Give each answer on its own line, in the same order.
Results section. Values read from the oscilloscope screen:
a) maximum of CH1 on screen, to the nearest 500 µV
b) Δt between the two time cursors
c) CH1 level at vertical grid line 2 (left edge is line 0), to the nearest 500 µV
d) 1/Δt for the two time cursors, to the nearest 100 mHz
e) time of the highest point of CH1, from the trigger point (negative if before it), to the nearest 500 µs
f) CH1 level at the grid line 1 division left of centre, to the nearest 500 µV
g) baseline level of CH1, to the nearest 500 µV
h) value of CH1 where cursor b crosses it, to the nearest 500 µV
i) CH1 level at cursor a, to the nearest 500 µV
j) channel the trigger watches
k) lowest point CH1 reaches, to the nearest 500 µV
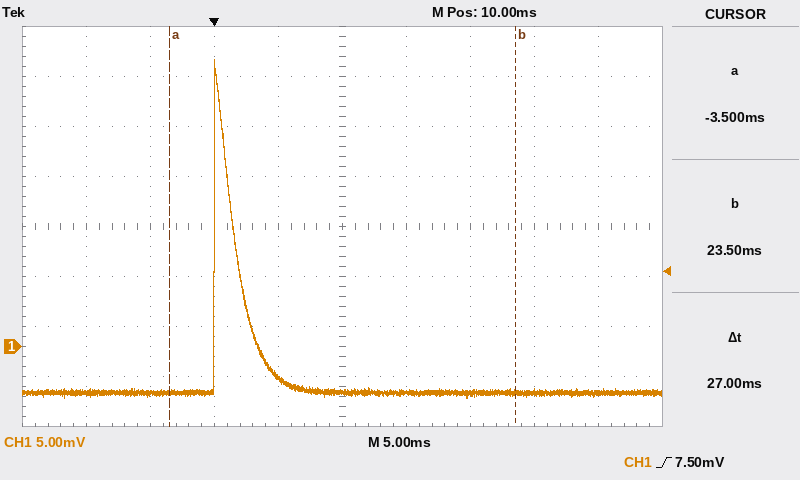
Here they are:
28.5 mV
27 ms
-4.5 mV
37.0 Hz
0.0 ms
-3.0 mV
-4.5 mV
-4.5 mV
-4.5 mV
CH1
-5.0 mV
